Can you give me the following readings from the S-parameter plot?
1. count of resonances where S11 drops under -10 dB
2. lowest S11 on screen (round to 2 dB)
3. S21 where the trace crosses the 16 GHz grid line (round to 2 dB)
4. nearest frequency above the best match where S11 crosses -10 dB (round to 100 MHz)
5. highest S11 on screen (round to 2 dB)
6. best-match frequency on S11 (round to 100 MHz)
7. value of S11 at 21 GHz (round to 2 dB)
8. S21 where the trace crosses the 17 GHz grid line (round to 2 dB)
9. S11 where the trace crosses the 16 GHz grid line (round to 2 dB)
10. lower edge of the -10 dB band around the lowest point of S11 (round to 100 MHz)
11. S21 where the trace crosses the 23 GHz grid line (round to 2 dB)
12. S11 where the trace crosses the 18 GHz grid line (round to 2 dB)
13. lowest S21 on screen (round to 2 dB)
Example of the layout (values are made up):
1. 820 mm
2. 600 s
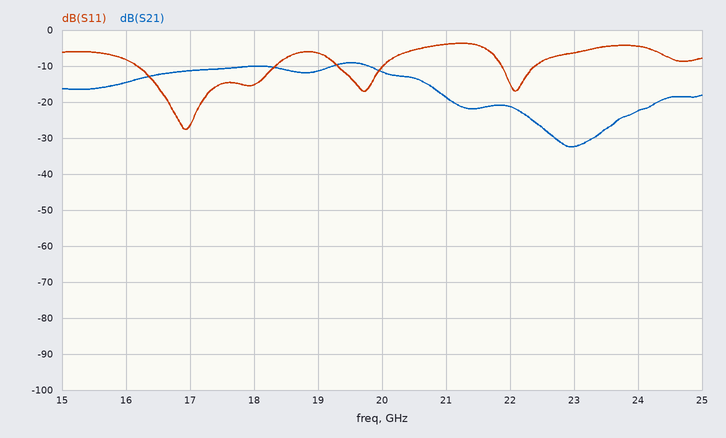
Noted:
1. 3
2. -28 dB
3. -14 dB
4. 18.3 GHz
5. -4 dB
6. 16.9 GHz
7. -4 dB
8. -12 dB
9. -8 dB
10. 16.2 GHz
11. -32 dB
12. -16 dB
13. -32 dB
